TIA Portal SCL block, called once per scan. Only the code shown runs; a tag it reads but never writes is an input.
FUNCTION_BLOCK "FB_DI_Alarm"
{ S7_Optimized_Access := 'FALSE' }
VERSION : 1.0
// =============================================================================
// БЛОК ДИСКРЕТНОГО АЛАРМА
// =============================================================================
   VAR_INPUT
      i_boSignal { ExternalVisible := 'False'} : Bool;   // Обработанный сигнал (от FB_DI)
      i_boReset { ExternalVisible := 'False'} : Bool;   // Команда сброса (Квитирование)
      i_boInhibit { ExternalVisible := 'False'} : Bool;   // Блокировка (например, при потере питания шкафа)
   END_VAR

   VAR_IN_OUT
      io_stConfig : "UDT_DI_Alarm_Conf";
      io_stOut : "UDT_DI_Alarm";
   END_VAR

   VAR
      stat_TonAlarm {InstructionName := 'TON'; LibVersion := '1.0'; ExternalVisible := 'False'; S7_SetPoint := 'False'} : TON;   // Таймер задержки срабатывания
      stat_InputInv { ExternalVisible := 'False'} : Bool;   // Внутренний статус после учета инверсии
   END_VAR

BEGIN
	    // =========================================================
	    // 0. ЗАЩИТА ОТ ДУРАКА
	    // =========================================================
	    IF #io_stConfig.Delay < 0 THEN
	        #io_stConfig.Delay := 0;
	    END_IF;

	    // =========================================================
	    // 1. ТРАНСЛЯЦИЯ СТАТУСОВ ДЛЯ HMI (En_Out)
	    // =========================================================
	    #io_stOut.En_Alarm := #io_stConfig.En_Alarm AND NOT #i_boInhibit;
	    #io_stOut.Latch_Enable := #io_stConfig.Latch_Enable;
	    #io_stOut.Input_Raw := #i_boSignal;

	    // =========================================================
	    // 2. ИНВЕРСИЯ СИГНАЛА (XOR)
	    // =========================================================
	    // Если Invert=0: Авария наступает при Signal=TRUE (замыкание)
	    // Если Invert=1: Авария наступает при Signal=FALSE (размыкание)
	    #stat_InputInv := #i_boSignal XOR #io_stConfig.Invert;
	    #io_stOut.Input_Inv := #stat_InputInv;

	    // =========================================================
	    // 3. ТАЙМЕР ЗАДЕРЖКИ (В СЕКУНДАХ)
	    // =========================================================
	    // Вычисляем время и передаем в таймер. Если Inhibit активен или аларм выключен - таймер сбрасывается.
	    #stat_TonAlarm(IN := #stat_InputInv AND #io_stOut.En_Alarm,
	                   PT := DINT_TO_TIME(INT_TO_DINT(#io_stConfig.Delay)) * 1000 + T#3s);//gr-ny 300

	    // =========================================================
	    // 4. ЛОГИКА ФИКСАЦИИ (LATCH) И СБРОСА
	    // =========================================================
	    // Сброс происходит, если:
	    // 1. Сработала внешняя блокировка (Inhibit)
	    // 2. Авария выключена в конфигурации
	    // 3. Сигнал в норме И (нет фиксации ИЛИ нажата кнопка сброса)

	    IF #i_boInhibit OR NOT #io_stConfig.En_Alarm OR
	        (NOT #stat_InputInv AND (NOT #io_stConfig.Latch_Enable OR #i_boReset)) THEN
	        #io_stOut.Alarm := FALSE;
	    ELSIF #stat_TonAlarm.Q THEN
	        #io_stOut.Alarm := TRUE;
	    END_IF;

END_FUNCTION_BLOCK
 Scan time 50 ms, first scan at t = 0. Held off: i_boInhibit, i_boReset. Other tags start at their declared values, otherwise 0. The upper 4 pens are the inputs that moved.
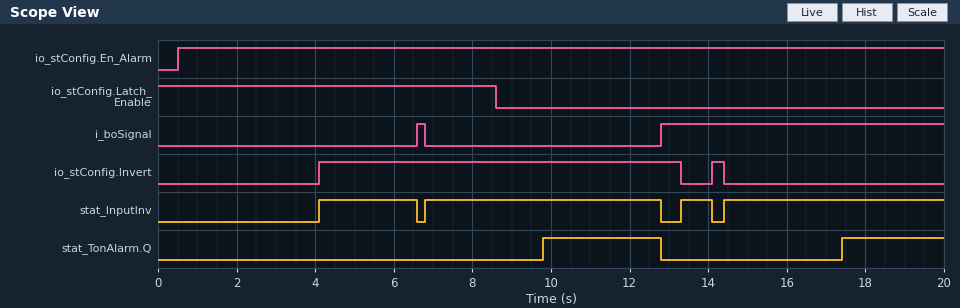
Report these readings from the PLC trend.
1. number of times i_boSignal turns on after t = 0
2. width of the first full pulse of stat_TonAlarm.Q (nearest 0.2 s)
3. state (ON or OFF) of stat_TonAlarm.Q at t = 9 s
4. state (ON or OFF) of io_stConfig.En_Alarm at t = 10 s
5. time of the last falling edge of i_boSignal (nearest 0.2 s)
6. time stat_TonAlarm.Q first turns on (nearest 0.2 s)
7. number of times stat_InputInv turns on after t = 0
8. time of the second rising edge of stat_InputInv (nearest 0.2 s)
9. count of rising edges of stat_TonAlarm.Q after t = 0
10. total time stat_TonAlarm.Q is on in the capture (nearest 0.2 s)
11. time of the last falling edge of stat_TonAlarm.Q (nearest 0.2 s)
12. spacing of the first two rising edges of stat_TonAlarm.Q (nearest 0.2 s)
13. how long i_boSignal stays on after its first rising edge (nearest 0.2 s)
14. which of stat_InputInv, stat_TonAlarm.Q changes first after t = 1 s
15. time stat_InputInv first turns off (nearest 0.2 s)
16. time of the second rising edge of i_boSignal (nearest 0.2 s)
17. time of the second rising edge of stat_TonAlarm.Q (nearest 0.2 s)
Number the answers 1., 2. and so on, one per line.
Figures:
1. 2
2. 3.0 s
3. OFF
4. ON
5. 6.8 s
6. 9.8 s
7. 4
8. 6.8 s
9. 2
10. 5.6 s
11. 12.8 s
12. 7.6 s
13. 0.2 s
14. stat_InputInv
15. 6.6 s
16. 12.8 s
17. 17.4 s
